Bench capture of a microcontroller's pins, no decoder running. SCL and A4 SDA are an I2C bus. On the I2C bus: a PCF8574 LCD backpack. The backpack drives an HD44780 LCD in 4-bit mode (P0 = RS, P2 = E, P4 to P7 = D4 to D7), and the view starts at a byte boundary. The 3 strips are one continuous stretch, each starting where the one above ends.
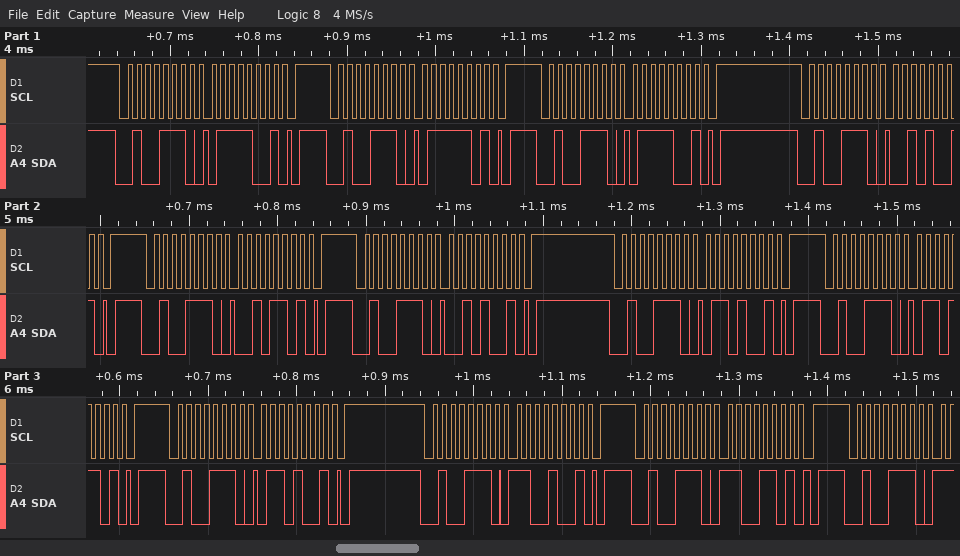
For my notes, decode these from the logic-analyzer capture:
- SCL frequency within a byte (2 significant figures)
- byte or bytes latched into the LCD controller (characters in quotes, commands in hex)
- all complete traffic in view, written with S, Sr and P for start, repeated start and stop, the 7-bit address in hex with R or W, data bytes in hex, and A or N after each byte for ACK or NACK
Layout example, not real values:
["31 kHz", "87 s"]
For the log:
["100 kHz", "'r'", "S 27W A 79 A P S 27W A 7D A P S 27W A 79 A P S 27W A 29 A P S 27W A 2D A P S 27W A 29 A P S 27W A 69 A P S 27W A 6D A P S 27W A 69 A P S 27W A C9 A P S 27W A CD A P S 27W A"]
